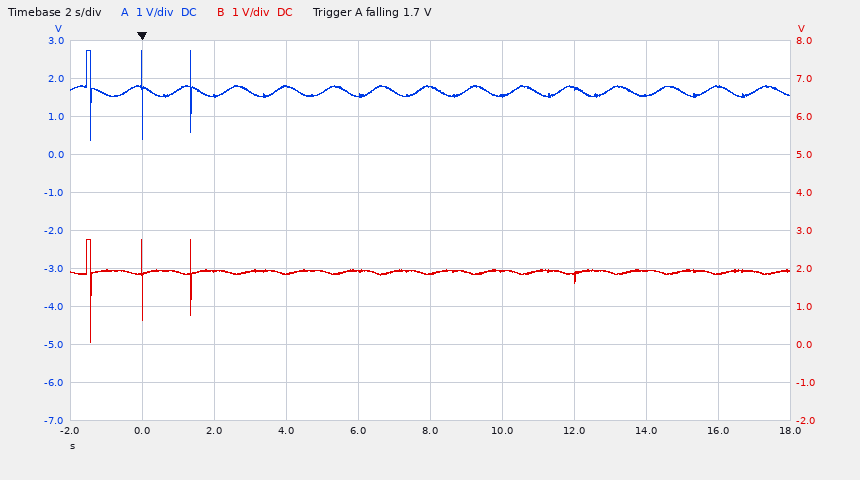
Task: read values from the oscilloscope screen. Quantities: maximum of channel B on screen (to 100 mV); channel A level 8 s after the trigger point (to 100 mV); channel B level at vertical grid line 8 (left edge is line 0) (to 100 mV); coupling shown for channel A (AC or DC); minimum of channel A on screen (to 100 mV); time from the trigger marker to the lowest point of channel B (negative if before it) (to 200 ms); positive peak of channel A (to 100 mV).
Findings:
2.8 V
1.8 V
1.9 V
DC
400 mV
-1.4 s
2.7 V
